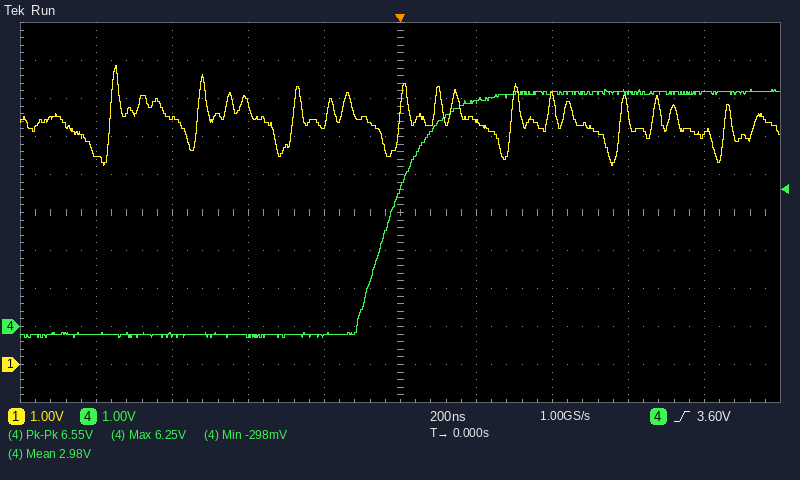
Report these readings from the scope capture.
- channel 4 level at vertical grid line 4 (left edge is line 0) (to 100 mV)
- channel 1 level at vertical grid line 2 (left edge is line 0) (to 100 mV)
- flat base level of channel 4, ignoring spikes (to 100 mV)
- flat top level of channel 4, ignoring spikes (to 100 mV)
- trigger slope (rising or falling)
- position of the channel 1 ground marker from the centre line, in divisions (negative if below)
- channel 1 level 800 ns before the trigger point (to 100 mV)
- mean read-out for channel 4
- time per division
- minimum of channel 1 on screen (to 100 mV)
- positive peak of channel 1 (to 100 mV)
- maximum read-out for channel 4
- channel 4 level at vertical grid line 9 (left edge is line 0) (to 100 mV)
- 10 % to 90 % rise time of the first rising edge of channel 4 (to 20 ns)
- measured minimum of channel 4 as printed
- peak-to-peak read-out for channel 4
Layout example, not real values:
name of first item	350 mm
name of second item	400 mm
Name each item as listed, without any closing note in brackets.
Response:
channel 4 level at vertical grid line 4 (left edge is line 0)	-200 mV
channel 1 level at vertical grid line 2 (left edge is line 0)	6.5 V
flat base level of channel 4, ignoring spikes	-200 mV
flat top level of channel 4, ignoring spikes	6.2 V
trigger slope	rising
position of the channel 1 ground marker from the centre line, in divisions	-4.0 div
channel 1 level 800 ns before the trigger point	5.6 V
mean read-out for channel 4	2.98 V
time per division	200 ns
minimum of channel 1 on screen	5.2 V
positive peak of channel 1	7.9 V
maximum read-out for channel 4	6.25 V
channel 4 level at vertical grid line 9 (left edge is line 0)	6.1 V
10 % to 90 % rise time of the first rising edge of channel 4	220 ns
measured minimum of channel 4 as printed	-298 mV
peak-to-peak read-out for channel 4	6.55 V
